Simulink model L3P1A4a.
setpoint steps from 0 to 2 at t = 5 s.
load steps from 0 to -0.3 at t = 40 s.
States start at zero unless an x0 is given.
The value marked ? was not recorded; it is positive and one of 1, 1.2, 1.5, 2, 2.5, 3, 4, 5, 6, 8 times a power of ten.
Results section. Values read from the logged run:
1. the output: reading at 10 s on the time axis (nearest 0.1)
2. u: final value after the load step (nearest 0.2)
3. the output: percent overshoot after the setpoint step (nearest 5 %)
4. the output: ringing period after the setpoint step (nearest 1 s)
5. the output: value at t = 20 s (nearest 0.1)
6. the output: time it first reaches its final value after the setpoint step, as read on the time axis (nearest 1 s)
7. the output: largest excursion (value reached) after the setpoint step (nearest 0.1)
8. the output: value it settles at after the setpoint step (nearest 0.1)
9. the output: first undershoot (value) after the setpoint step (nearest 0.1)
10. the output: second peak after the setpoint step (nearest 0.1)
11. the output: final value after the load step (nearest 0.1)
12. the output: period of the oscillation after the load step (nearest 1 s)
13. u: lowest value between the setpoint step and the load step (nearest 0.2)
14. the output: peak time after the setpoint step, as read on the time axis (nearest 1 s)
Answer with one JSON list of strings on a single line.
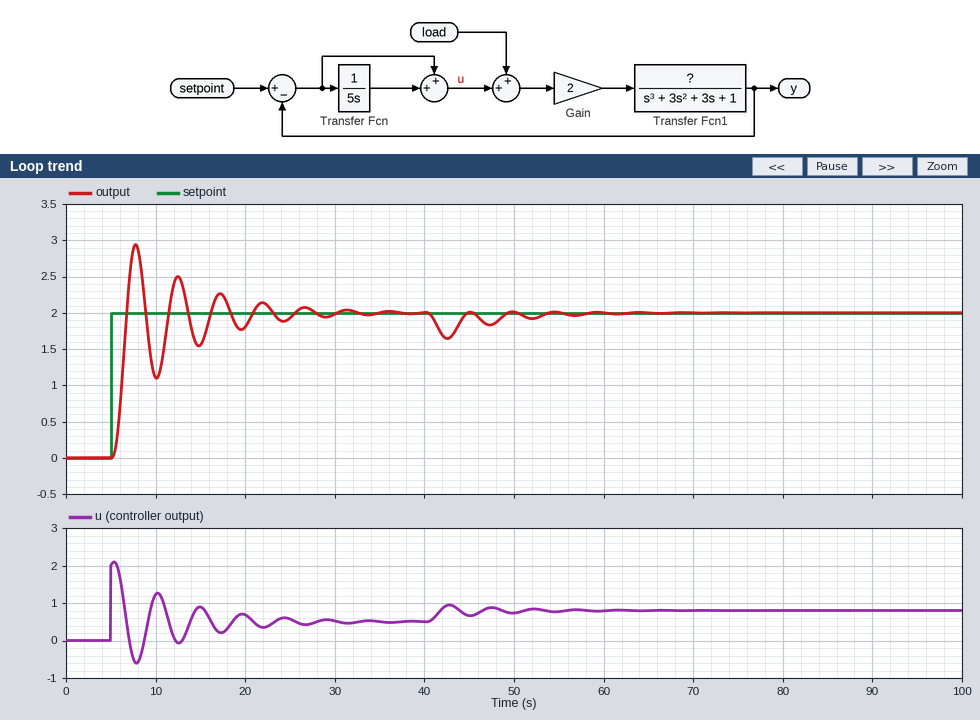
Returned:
["1.1", "0.8", "45 %", "5 s", "1.8", "7 s", "2.9", "2.0", "1.1", "2.5", "2.0", "5 s", "-0.6", "8 s"]
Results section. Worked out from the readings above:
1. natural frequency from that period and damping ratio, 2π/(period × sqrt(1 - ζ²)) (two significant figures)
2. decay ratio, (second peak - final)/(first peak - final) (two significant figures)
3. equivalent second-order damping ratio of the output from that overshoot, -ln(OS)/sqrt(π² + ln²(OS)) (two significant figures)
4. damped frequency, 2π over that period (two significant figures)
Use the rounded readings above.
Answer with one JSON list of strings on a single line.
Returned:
["1.3 rad/s", "0.56", "0.25", "1.3 rad/s"]
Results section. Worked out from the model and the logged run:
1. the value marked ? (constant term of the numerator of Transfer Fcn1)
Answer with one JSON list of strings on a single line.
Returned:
["2"]
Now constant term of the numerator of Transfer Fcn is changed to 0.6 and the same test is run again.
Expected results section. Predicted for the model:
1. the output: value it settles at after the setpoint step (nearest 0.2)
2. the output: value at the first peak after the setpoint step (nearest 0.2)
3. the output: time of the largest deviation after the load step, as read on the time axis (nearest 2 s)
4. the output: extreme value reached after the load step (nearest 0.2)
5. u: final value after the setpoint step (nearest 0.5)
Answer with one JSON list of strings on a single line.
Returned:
["2.0", "2.8", "42 s", "1.6", "0.5"]
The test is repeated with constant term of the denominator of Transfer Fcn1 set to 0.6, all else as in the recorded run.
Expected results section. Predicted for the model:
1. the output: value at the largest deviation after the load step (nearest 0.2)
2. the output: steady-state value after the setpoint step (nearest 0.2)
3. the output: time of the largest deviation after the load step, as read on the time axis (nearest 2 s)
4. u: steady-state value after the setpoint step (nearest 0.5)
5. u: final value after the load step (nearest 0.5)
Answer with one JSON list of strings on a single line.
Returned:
["1.6", "2.0", "42 s", "0.5", "0.5"]
